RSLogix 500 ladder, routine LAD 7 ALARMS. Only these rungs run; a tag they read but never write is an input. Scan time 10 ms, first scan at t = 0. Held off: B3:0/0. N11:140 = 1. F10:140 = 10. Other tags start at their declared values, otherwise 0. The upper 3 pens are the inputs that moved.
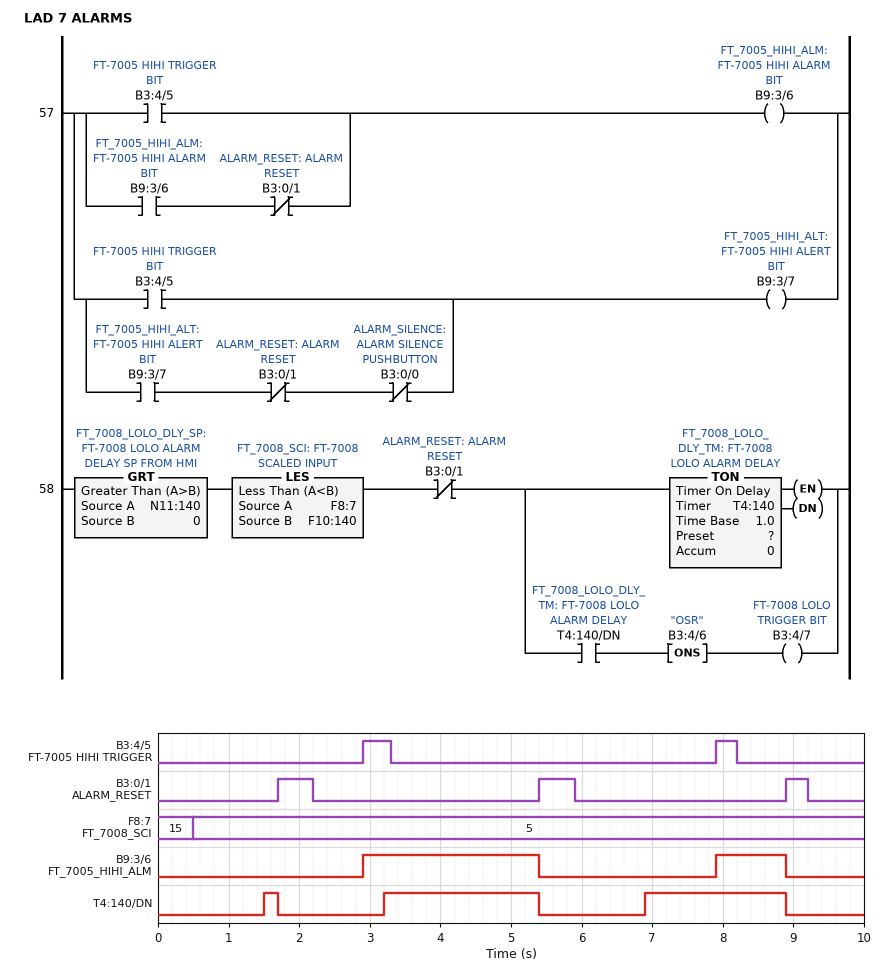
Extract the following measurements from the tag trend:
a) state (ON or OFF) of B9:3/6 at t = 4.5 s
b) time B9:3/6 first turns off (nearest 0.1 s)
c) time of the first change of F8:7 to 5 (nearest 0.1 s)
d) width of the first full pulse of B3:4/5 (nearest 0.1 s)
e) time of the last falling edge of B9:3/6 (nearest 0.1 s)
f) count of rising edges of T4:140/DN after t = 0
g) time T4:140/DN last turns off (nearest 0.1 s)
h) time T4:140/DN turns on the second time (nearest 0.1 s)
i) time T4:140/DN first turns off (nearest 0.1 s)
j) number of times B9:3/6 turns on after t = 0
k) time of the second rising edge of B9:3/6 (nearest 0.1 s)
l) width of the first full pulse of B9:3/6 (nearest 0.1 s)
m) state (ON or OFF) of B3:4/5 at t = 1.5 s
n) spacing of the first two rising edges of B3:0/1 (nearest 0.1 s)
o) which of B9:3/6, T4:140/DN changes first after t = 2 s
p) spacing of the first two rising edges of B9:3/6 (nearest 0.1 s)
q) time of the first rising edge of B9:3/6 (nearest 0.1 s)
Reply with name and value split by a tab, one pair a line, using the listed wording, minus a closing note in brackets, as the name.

state (ON or OFF) of B9:3/6 at t = 4.5 s	ON
time B9:3/6 first turns off	5.4 s
time of the first change of F8:7 to 5	0.5 s
width of the first full pulse of B3:4/5	0.4 s
time of the last falling edge of B9:3/6	8.9 s
count of rising edges of T4:140/DN after t = 0	3
time T4:140/DN last turns off	8.9 s
time T4:140/DN turns on the second time	3.2 s
time T4:140/DN first turns off	1.7 s
number of times B9:3/6 turns on after t = 0	2
time of the second rising edge of B9:3/6	7.9 s
width of the first full pulse of B9:3/6	2.5 s
state (ON or OFF) of B3:4/5 at t = 1.5 s	OFF
spacing of the first two rising edges of B3:0/1	3.7 s
which of B9:3/6, T4:140/DN changes first after t = 2 s	B9:3/6
spacing of the first two rising edges of B9:3/6	5.0 s
time of the first rising edge of B9:3/6	2.9 s
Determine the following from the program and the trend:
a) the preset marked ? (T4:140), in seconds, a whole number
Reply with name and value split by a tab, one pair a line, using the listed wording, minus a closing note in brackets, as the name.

the preset marked ? (T4:140), in seconds, a whole number	1 s
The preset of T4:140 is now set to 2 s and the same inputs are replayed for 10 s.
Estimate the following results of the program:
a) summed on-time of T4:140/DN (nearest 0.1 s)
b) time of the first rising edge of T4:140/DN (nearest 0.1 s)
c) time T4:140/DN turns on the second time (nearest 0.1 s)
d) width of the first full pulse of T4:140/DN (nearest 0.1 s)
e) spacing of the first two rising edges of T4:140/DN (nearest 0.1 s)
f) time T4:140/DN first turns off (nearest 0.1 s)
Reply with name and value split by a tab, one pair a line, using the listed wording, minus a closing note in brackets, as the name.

summed on-time of T4:140/DN	2.2 s
time of the first rising edge of T4:140/DN	4.2 s
time T4:140/DN turns on the second time	7.9 s
width of the first full pulse of T4:140/DN	1.2 s
spacing of the first two rising edges of T4:140/DN	3.7 s
time T4:140/DN first turns off	5.4 s
